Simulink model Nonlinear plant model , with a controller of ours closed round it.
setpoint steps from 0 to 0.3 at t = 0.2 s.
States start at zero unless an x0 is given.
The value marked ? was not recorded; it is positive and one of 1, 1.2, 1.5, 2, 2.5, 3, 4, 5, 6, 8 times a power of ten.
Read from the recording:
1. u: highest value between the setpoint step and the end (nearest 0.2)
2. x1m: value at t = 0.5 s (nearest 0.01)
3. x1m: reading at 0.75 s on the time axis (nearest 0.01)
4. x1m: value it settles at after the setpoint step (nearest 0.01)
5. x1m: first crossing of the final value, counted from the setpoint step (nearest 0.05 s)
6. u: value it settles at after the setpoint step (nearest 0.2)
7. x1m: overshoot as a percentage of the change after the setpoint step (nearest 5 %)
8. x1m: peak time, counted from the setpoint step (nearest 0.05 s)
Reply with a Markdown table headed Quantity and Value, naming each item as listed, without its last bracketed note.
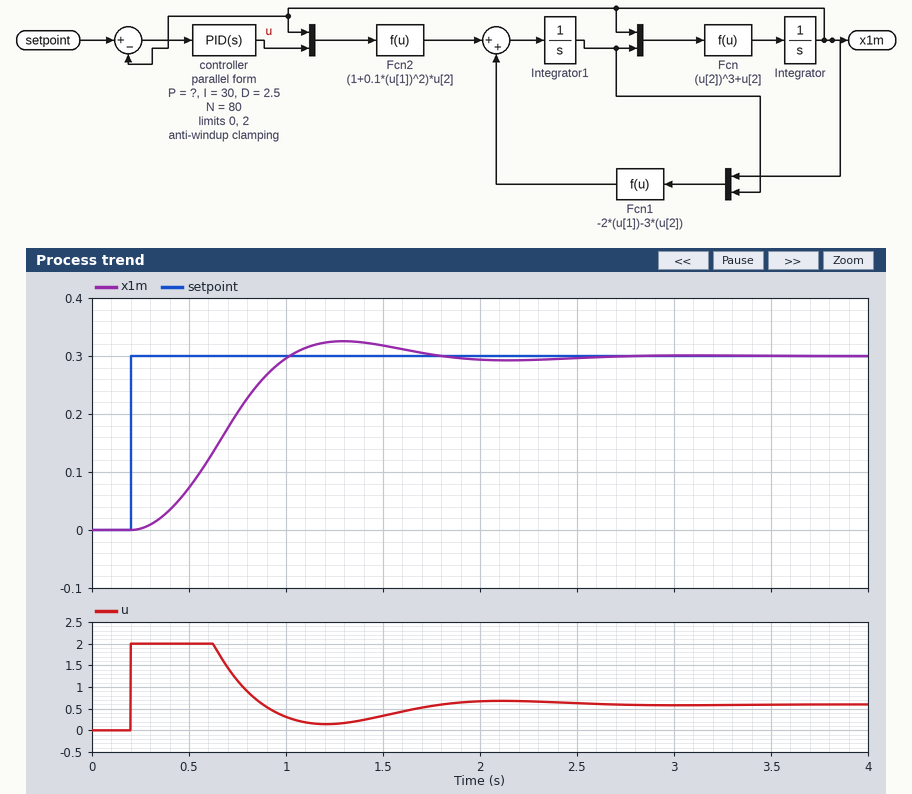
| Quantity | Value |
|---|---|
| u: highest value between the setpoint step and the end | 2.0 |
| x1m: value at t = 0.5 s | 0.07 |
| x1m: reading at 0.75 s on the time axis | 0.20 |
| x1m: value it settles at after the setpoint step | 0.30 |
| x1m: first crossing of the final value, counted from the setpoint step | 0.80 s |
| u: value it settles at after the setpoint step | 0.6 |
| x1m: overshoot as a percentage of the change after the setpoint step | 10 % |
| x1m: peak time, counted from the setpoint step | 1.10 s |
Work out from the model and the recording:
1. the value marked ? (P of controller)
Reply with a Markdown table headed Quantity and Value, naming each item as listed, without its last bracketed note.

| Quantity | Value |
|---|---|
| the value marked ? | 20 |
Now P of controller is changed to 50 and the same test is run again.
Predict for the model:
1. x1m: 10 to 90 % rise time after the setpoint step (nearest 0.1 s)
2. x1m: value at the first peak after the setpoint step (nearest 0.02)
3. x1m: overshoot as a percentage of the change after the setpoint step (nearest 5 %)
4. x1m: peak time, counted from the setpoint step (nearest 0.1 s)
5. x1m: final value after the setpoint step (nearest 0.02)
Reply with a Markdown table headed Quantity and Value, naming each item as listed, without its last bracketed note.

| Quantity | Value |
|---|---|
| x1m: 10 to 90 % rise time after the setpoint step | 0.5 s |
| x1m: value at the first peak after the setpoint step | 0.34 |
| x1m: overshoot as a percentage of the change after the setpoint step | 15 % |
| x1m: peak time, counted from the setpoint step | 1.0 s |
| x1m: final value after the setpoint step | 0.30 |
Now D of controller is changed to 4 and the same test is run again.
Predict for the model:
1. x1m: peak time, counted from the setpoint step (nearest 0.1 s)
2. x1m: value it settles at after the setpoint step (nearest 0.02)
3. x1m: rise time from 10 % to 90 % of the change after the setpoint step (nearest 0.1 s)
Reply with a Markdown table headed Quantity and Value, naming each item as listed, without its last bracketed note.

| Quantity | Value |
|---|---|
| x1m: peak time, counted from the setpoint step | 1.3 s |
| x1m: value it settles at after the setpoint step | 0.30 |
| x1m: rise time from 10 % to 90 % of the change after the setpoint step | 0.6 s |
